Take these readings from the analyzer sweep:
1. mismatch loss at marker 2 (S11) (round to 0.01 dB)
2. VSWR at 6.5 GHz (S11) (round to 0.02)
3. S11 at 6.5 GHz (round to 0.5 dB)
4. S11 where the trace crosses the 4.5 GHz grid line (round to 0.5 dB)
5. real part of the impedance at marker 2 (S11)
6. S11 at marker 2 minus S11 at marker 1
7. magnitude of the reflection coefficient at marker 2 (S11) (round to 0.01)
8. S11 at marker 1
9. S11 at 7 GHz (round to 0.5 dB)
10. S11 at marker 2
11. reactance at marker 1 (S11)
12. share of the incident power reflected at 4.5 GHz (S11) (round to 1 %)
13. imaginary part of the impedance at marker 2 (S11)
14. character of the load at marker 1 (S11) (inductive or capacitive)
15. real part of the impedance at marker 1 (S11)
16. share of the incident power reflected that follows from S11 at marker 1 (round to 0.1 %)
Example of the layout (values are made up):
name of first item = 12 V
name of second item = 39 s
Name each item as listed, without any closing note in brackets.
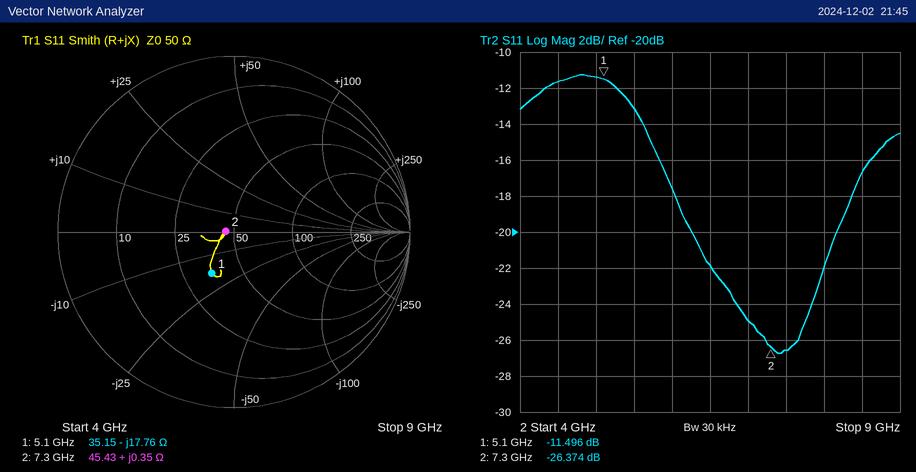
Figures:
mismatch loss at marker 2 (S11) = 0.01 dB
VSWR at 6.5 GHz (S11) = 1.18
S11 at 6.5 GHz = -22.0 dB
S11 where the trace crosses the 4.5 GHz grid line = -11.5 dB
real part of the impedance at marker 2 = 45.43 Ω
S11 at marker 2 minus S11 at marker 1 = -14.878 dB
magnitude of the reflection coefficient at marker 2 (S11) = 0.05
S11 at marker 1 = -11.496 dB
S11 at 7 GHz = -25.0 dB
S11 at marker 2 = -26.374 dB
reactance at marker 1 = -17.76 Ω
share of the incident power reflected at 4.5 GHz (S11) = 7 %
imaginary part of the impedance at marker 2 = +0.35 Ω
character of the load at marker 1 (S11) = capacitive
real part of the impedance at marker 1 = 35.15 Ω
share of the incident power reflected that follows from S11 at marker 1 = 7.1 %
